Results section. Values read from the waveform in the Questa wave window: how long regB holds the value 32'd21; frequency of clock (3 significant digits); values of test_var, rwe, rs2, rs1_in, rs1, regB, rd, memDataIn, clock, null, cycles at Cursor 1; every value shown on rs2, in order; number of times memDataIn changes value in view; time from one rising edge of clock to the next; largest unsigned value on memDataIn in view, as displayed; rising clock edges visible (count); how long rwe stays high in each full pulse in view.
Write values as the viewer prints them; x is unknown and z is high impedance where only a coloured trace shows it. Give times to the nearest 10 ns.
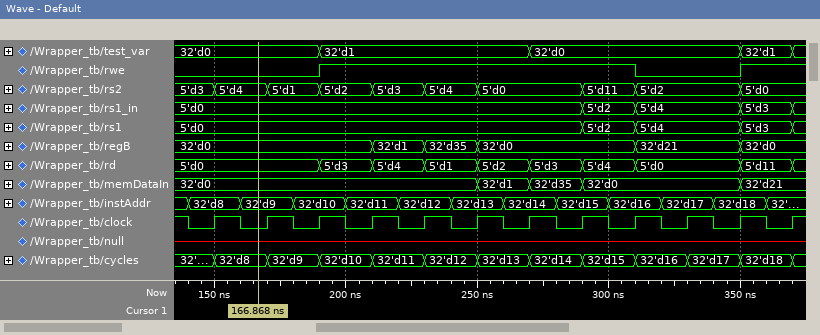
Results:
40 ns
50.0 MHz
test_var=32'd0, rwe=0, rs2=5'd4, rs1_in=5'd0, rs1=5'd0, regB=32'd0, rd=5'd0, memDataIn=32'd0, clock=0, null=x, cycles=32'd8
5'd3, 5'd4, 5'd1, 5'd2, 5'd3, 5'd4, 5'd0, 5'd11, 5'd2, 5'd0
4
20 ns
32'd35
12
120 ns
